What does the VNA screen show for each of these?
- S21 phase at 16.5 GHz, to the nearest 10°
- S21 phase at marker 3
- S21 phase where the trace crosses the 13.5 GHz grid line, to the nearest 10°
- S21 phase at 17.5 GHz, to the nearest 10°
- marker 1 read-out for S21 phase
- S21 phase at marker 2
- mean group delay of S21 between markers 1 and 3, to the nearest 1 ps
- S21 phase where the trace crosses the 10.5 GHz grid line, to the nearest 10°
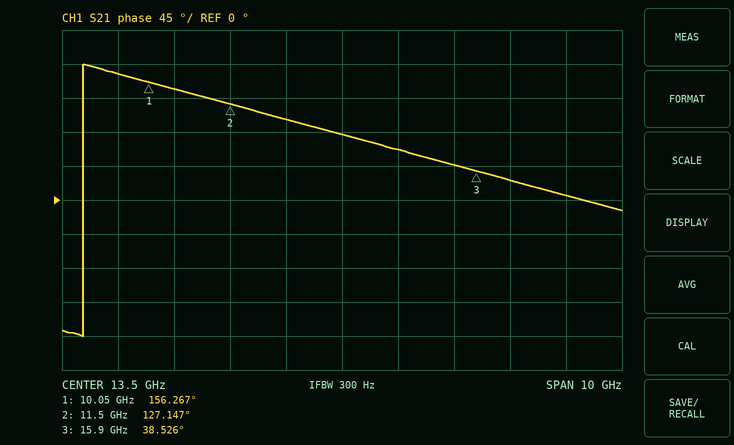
30°
38.526°
90°
10°
156.267°
127.147°
56 ps
150°
